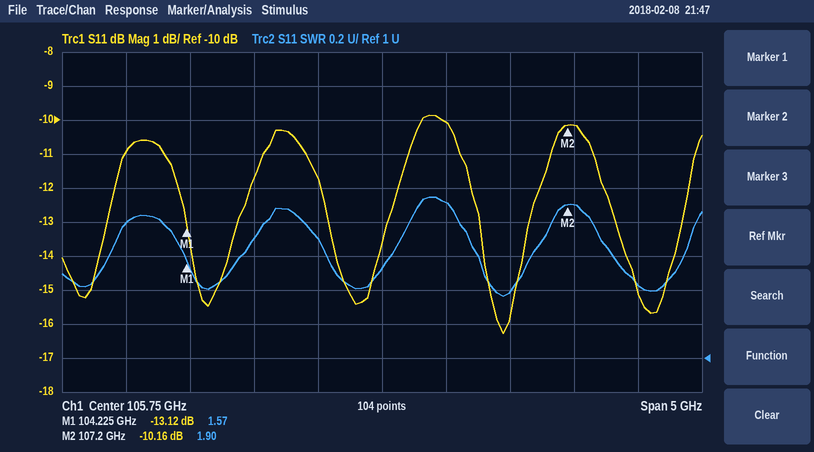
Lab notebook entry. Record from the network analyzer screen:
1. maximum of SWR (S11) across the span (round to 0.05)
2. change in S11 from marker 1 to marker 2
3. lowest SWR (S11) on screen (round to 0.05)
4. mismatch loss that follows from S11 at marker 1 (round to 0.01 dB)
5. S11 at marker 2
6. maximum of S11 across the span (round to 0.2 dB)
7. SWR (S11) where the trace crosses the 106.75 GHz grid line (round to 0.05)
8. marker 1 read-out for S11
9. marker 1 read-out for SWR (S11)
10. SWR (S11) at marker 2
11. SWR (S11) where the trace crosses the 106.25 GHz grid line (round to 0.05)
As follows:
1.95
2.96 dB
1.35
0.22 dB
-10.16 dB
-9.8 dB
1.40
-13.12 dB
1.57
1.90
1.90
